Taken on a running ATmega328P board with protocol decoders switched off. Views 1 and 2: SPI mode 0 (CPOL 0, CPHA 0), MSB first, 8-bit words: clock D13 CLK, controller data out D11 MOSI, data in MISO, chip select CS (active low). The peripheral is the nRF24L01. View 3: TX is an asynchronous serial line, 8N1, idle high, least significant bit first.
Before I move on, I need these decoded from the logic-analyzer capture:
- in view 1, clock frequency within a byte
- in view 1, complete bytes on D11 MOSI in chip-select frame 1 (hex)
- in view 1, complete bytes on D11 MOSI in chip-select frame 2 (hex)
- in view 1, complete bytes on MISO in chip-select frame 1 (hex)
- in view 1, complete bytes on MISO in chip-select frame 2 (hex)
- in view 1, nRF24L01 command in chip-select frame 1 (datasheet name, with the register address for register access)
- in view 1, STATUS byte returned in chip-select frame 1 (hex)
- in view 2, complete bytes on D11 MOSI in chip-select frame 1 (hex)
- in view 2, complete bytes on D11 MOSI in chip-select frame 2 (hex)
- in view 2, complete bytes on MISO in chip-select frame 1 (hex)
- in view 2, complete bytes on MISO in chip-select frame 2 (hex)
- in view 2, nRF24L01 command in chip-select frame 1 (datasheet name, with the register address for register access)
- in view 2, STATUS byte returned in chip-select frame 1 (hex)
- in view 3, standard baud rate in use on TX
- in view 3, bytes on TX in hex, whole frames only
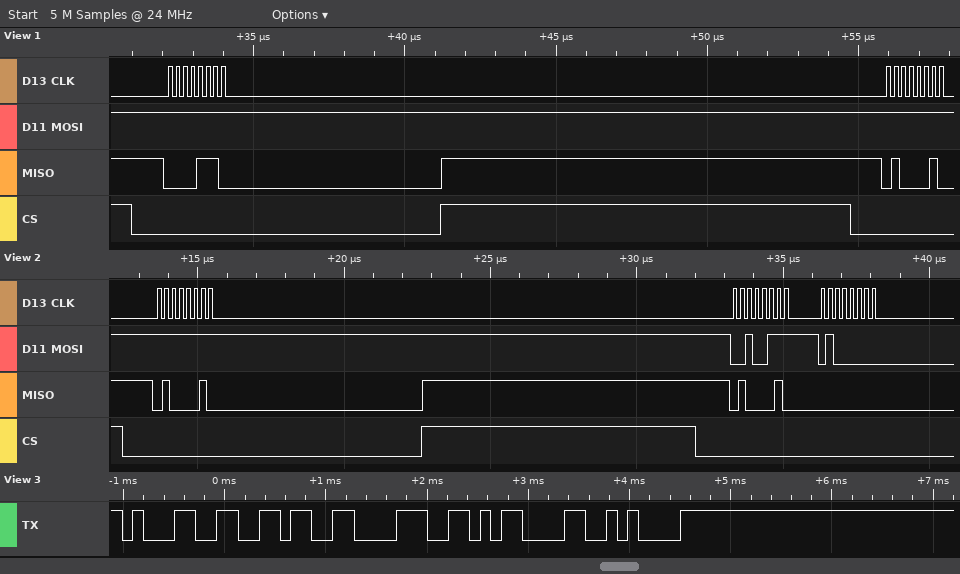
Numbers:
4 MHz
0xFF
0xFF
0x0E
0x42
NOP
0x0E
0xFF
0x27 0x40
0x42
0x42 0x00
NOP
0x42
9600 baud
0x31 0x36 0x38 0x0D 0x0A
